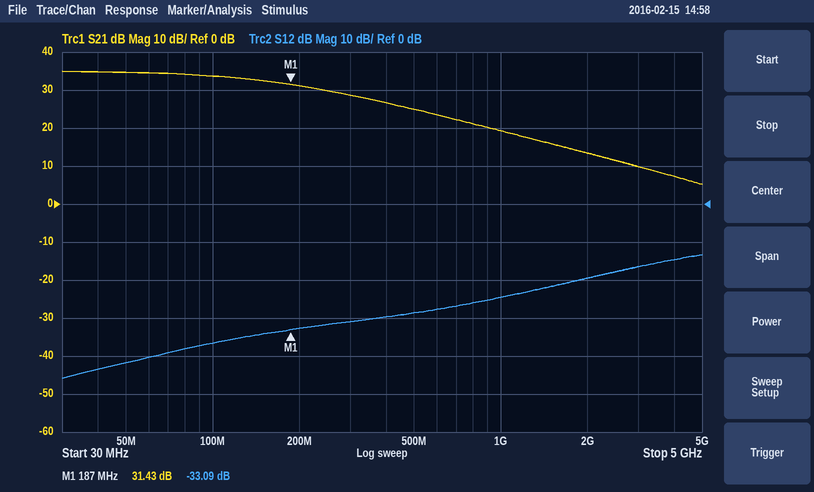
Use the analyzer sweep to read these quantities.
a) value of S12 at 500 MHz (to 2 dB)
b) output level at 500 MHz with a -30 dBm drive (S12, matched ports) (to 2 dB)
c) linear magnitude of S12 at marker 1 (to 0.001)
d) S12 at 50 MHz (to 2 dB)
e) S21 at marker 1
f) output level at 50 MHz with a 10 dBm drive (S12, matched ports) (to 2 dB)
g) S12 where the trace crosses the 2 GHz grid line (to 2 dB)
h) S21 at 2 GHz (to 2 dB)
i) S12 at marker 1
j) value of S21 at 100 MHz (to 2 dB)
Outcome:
-28 dB
-58 dBm
0.022
-42 dB
31.43 dB
-32 dBm
-20 dB
14 dB
-33.09 dB
34 dB
